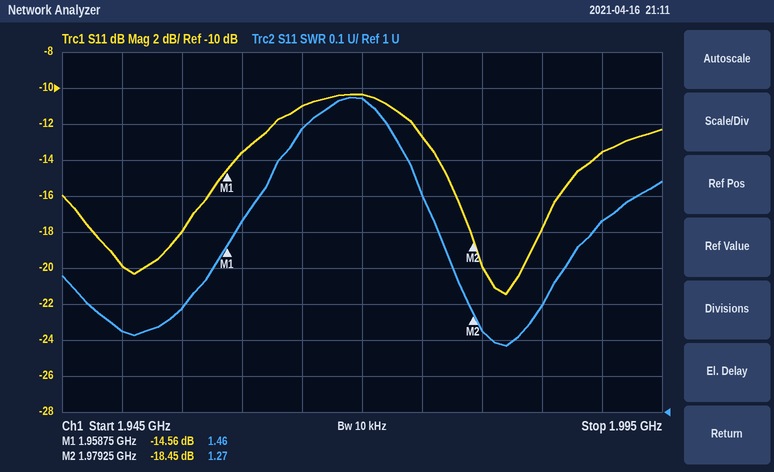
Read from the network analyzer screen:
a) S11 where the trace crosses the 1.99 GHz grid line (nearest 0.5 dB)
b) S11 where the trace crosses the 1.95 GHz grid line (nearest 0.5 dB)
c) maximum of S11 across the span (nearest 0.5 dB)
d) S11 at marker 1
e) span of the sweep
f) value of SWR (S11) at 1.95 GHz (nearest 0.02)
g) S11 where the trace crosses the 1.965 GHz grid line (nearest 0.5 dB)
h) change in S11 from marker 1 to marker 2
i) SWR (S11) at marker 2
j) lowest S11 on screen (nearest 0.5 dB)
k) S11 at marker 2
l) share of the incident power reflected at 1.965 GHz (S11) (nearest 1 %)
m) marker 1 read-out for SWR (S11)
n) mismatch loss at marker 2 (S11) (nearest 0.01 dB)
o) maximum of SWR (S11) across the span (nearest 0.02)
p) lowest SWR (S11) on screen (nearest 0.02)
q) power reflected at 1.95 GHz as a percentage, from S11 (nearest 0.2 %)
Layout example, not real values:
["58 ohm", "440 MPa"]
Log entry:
["-13.5 dB", "-20.0 dB", "-10.5 dB", "-14.56 dB", "50 MHz", "1.22", "-11.0 dB", "-3.89 dB", "1.27", "-21.5 dB", "-18.45 dB", "8 %", "1.46", "0.06 dB", "1.88", "1.18", "1.0 %"]
